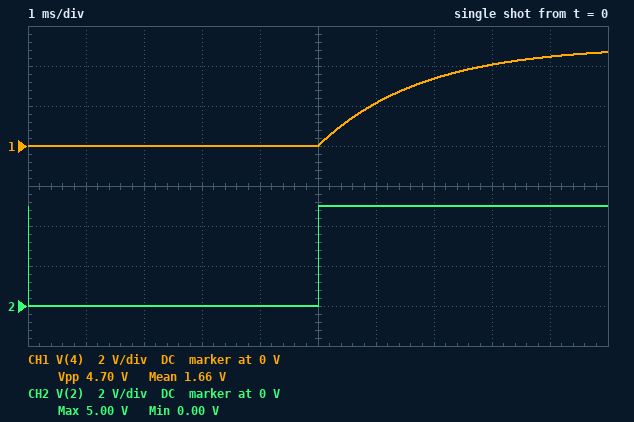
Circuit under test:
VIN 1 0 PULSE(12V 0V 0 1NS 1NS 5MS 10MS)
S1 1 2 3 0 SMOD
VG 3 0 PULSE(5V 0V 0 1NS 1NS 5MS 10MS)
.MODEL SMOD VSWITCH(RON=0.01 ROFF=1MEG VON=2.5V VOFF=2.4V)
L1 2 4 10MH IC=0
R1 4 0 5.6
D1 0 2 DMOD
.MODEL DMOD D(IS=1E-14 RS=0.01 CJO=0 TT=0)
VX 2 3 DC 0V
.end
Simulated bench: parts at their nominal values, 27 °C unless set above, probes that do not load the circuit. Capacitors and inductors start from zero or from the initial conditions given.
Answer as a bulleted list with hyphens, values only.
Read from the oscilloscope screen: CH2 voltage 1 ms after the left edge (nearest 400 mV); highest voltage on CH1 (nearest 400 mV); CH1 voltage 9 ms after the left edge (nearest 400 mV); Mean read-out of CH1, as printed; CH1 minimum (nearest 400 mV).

- 0 V
- 4.8 V
- 4.4 V
- 1.66 V
- 0 V
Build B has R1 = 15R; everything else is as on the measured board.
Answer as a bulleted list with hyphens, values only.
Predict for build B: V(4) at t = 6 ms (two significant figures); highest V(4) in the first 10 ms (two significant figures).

- 3.9 V
- 5.0 V
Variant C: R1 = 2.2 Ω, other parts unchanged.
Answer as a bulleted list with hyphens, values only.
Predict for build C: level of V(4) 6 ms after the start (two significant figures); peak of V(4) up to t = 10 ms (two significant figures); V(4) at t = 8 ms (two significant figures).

- 990 mV
- 3.3 V
- 2.4 V
